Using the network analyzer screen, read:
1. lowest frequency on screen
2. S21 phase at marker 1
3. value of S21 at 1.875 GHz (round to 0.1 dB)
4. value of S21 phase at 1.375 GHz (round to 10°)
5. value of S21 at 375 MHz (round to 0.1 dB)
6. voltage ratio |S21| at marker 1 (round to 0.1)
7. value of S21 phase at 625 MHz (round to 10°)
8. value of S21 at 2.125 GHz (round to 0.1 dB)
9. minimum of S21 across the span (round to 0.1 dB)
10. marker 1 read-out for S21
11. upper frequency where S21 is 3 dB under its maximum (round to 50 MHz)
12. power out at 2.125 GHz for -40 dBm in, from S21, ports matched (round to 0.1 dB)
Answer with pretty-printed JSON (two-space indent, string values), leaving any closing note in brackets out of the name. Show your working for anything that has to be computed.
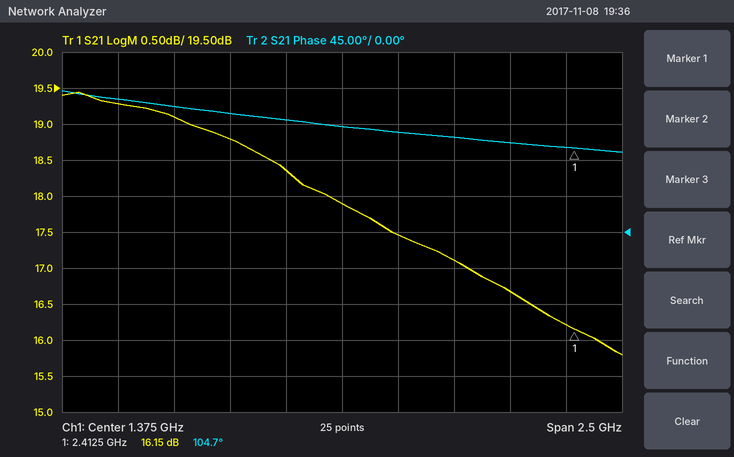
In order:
{
  "lowest frequency on screen": "125 MHz",
  "S21 phase at marker 1": "104.7°",
  "value of S21 at 1.875 GHz": "17.1 dB",
  "value of S21 phase at 1.375 GHz": "130°",
  "value of S21 at 375 MHz": "19.3 dB",
  "voltage ratio |S21| at marker 1": "10^(16.15/20) ≈ 6.4",
  "value of S21 phase at 625 MHz": "160°",
  "value of S21 at 2.125 GHz": "16.7 dB",
  "minimum of S21 across the span": "15.8 dB",
  "marker 1 read-out for S21": "16.15 dB",
  "upper frequency where S21 is 3 dB under its maximum": "2.25 GHz",
  "power out at 2.125 GHz for -40 dBm in, from S21, ports matched": "-40 dBm + (16.7 dB) = -23.3 dBm"
}
